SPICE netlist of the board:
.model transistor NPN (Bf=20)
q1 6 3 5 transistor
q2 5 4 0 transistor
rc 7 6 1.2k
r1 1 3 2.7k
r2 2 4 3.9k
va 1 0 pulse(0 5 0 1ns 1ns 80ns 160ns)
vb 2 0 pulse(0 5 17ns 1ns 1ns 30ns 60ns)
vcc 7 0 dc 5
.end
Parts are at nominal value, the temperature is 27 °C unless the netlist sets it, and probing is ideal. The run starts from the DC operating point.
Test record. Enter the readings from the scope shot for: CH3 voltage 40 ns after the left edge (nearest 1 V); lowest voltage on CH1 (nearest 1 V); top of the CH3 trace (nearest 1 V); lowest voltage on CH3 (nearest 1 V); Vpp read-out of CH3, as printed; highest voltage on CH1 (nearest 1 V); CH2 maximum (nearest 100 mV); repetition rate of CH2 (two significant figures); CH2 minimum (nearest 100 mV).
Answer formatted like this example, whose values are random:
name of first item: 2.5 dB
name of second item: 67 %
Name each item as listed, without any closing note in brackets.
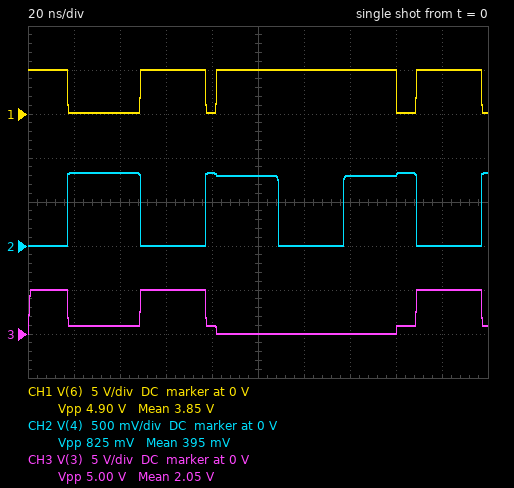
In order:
CH3 voltage 40 ns after the left edge: 1 V
lowest voltage on CH1: 0 V
top of the CH3 trace: 5 V
lowest voltage on CH3: 0 V
Vpp read-out of CH3, as printed: 5.00 V
highest voltage on CH1: 5 V
CH2 maximum: 800 mV
repetition rate of CH2: 17 MHz
CH2 minimum: 0 V
